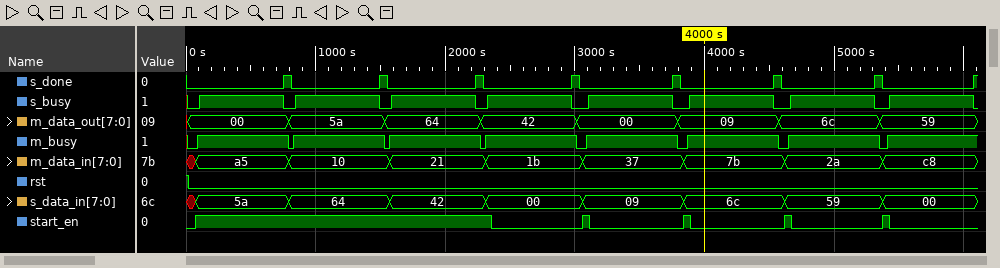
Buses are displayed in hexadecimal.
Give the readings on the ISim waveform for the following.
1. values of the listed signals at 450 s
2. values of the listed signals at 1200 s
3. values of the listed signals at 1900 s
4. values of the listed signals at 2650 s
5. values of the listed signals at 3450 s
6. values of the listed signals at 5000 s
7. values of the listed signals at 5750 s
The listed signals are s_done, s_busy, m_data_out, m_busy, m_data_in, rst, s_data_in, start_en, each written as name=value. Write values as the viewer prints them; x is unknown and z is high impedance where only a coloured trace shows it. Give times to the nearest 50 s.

s_done=0, s_busy=1, m_data_out=00, m_busy=1, m_data_in=a5, rst=0, s_data_in=5a, start_en=1
s_done=0, s_busy=1, m_data_out=5a, m_busy=1, m_data_in=10, rst=0, s_data_in=64, start_en=1
s_done=0, s_busy=1, m_data_out=64, m_busy=1, m_data_in=21, rst=0, s_data_in=42, start_en=1
s_done=0, s_busy=1, m_data_out=42, m_busy=1, m_data_in=1b, rst=0, s_data_in=00, start_en=0
s_done=0, s_busy=1, m_data_out=00, m_busy=1, m_data_in=37, rst=0, s_data_in=09, start_en=0
s_done=0, s_busy=1, m_data_out=6c, m_busy=1, m_data_in=2a, rst=0, s_data_in=59, start_en=0
s_done=0, s_busy=1, m_data_out=59, m_busy=1, m_data_in=c8, rst=0, s_data_in=00, start_en=0
